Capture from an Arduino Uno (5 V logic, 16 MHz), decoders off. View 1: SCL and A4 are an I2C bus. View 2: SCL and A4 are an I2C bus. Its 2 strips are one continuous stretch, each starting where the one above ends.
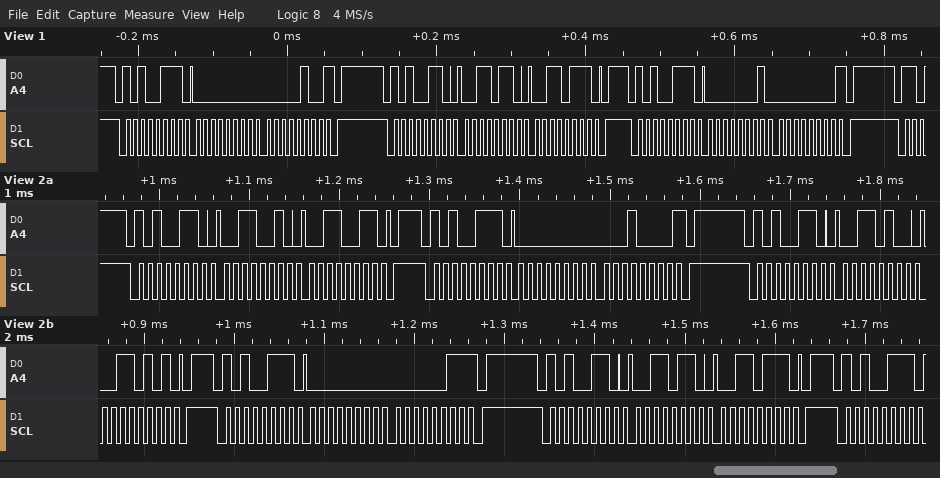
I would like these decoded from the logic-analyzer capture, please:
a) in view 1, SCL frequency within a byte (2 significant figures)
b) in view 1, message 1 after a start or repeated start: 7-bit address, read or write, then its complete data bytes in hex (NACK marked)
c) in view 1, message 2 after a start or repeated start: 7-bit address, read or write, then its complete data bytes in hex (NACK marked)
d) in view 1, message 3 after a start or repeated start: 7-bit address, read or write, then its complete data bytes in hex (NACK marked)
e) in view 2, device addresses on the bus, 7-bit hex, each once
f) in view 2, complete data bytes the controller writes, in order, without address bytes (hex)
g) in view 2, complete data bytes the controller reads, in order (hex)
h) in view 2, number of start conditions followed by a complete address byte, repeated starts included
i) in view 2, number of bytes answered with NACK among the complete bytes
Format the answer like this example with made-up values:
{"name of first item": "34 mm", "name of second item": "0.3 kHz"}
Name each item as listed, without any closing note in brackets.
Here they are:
{"in view 1, SCL frequency within a byte": "100 kHz", "in view 1, message 1 after a start or repeated start: 7-bit address, read or write, then its complete data bytes in hex": "0x53 read: 00 04 NACK", "in view 1, message 2 after a start or repeated start: 7-bit address, read or write, then its complete data bytes in hex": "0x53 write: 36 37", "in view 1, message 3 after a start or repeated start: 7-bit address, read or write, then its complete data bytes in hex": "0x53 read: 01 00 NACK", "in view 2, device addresses on the bus, 7-bit hex, each once": "0x53", "in view 2, complete data bytes the controller writes, in order, without address bytes": "32 33 34 35 36 37", "in view 2, complete data bytes the controller reads, in order": "00 10 00 03", "in view 2, number of start conditions followed by a complete address byte, repeated starts included": "6", "in view 2, number of bytes answered with NACK among the complete bytes": "2"}
